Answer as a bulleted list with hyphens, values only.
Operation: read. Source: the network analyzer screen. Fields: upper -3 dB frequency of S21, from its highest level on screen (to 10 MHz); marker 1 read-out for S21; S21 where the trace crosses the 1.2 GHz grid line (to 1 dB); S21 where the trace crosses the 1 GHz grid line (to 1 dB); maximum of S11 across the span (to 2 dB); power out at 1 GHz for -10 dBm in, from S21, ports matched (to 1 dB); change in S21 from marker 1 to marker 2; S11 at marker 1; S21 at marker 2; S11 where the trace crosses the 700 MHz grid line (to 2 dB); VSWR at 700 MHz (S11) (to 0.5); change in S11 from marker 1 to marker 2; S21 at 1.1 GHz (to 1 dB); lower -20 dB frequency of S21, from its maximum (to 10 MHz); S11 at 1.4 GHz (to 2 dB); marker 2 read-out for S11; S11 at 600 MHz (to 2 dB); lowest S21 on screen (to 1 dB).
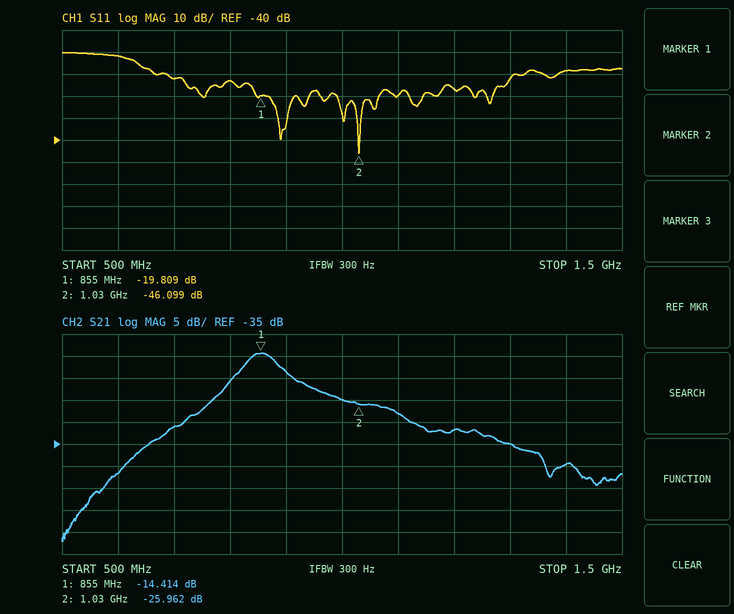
- 890 MHz
- -14.414 dB
- -32 dB
- -25 dB
- 0 dB
- -35 dBm
- -11.548 dB
- -19.809 dB
- -25.962 dB
- -12 dB
- 1.5
- -26.290 dB
- -28 dB
- 660 MHz
- -8 dB
- -46.099 dB
- -2 dB
- -57 dB
